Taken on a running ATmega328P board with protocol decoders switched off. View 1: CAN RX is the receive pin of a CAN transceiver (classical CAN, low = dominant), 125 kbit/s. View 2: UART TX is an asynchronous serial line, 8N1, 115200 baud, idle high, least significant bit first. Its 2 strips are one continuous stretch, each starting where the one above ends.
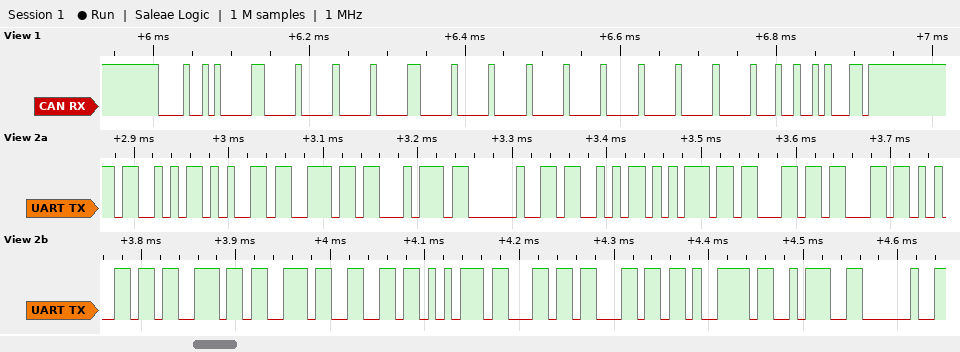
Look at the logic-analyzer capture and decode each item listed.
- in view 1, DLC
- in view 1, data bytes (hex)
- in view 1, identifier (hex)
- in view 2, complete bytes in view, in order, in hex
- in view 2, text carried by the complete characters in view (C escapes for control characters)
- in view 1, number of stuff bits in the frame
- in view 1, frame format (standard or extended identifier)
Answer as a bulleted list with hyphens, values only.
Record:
- 8
- 00 00 40 00 00 00 00 00
- 0x094
- 53 65 6E 74 20 53 75 63 63 65 73 73 66 75 6C 6C 79 3A 20
- "Sent Successfully: "
- 14
- standard
